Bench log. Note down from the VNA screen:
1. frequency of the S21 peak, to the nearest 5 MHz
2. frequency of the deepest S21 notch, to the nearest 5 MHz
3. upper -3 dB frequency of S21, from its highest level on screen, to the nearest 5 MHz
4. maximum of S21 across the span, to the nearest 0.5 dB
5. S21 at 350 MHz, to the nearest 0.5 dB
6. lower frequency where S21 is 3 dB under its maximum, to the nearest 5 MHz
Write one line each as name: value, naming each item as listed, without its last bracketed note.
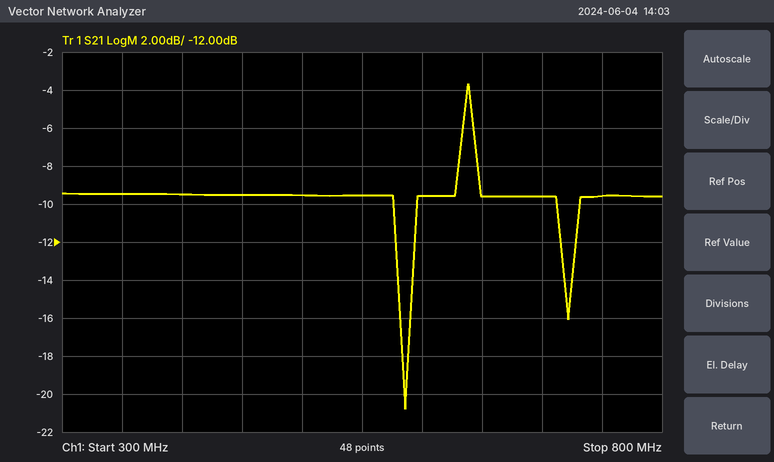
frequency of the S21 peak, to the nearest 5 MHz: 640 MHz
frequency of the deepest S21 notch, to the nearest 5 MHz: 585 MHz
upper -3 dB frequency of S21, from its highest level on screen, to the nearest 5 MHz: 645 MHz
maximum of S21 across the span, to the nearest 0.5 dB: -3.5 dB
S21 at 350 MHz, to the nearest 0.5 dB: -9.5 dB
lower frequency where S21 is 3 dB under its maximum, to the nearest 5 MHz: 635 MHz
